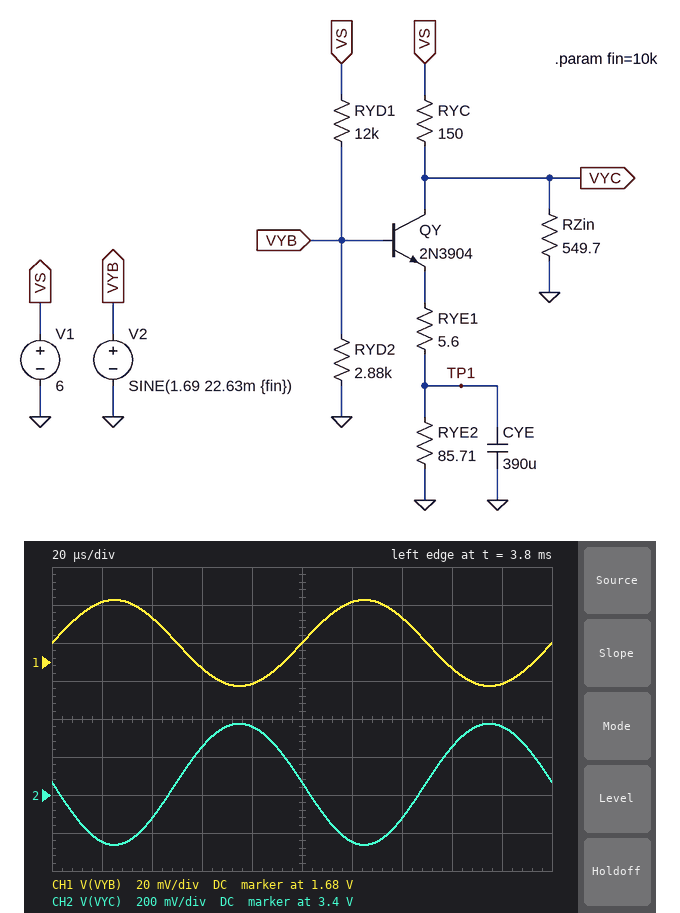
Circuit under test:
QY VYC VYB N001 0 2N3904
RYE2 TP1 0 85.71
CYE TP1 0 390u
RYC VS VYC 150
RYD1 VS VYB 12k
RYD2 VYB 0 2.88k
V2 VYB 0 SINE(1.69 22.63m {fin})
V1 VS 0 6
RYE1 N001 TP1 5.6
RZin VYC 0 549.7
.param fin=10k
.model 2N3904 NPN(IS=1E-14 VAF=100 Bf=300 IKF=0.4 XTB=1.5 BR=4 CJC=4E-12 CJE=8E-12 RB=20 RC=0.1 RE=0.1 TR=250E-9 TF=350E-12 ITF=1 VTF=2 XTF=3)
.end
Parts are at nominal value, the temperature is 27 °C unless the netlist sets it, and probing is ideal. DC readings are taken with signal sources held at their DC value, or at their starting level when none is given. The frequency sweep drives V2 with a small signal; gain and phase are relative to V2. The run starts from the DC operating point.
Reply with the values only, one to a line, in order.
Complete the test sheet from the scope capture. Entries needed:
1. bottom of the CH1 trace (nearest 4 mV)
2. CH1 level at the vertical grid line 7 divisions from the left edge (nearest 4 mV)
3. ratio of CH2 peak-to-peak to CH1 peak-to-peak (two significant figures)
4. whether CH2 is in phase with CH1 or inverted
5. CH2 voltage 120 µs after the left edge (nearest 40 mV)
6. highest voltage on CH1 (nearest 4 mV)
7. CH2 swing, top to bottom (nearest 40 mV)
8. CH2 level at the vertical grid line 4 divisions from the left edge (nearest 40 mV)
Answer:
1.668 V
1.704 V
14
inverted
3.16 V
1.712 V
640 mV
3.76 V
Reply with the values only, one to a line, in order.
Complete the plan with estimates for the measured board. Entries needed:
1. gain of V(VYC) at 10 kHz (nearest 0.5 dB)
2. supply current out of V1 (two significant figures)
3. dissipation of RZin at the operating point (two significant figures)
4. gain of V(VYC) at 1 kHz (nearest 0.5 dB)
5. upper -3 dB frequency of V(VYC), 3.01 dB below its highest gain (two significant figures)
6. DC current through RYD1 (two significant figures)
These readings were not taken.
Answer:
23.0 dB
17 mA
22 mW
23.0 dB
74 MHz
360 µA
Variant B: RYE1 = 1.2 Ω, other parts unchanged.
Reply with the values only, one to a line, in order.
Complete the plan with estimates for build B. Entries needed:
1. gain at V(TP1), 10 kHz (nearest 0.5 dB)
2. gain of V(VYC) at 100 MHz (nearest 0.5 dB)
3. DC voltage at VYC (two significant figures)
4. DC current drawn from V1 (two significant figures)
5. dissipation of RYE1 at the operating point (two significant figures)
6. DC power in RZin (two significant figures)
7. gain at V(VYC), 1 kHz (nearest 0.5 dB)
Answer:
-39.5 dB
21.0 dB
3.4 V
18 mA
150 µW
21 mW
30.0 dB
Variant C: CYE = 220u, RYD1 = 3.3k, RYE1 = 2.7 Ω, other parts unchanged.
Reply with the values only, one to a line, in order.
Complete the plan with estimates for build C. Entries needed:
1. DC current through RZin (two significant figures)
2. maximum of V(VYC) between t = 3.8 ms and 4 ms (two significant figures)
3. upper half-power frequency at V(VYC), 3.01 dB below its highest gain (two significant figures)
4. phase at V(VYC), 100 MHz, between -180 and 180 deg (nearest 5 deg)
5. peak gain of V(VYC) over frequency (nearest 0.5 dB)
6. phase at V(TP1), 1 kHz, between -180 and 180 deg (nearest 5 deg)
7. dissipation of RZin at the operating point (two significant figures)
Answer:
6.2 mA
3.9 V
53 MHz
110 deg
27.0 dB
-80 deg
21 mW
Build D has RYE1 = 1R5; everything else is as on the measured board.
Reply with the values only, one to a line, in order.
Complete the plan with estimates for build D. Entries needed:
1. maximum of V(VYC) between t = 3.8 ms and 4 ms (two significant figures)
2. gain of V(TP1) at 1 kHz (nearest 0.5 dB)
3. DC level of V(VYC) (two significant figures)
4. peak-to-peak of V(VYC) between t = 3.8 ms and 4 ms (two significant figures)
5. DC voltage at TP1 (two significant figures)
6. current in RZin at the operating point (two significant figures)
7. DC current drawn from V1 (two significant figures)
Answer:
4.0 V
-20.0 dB
3.4 V
1.3 V
950 mV
6.2 mA
18 mA
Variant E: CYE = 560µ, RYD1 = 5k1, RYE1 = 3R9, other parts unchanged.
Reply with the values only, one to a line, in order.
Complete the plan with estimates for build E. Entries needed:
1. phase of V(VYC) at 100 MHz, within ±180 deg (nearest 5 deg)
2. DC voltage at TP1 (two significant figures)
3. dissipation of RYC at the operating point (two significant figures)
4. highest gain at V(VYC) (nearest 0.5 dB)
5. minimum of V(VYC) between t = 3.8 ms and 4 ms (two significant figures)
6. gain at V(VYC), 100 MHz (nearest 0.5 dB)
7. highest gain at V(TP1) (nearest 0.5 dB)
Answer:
115 deg
930 mV
44 mW
25.0 dB
3.0 V
19.5 dB
-0.5 dB
